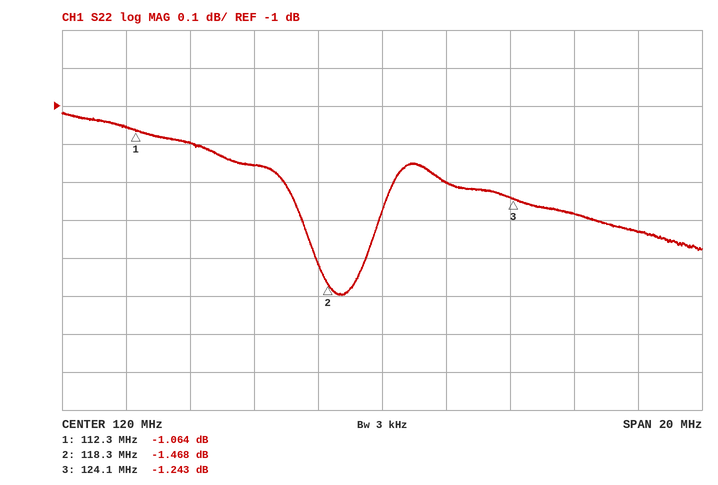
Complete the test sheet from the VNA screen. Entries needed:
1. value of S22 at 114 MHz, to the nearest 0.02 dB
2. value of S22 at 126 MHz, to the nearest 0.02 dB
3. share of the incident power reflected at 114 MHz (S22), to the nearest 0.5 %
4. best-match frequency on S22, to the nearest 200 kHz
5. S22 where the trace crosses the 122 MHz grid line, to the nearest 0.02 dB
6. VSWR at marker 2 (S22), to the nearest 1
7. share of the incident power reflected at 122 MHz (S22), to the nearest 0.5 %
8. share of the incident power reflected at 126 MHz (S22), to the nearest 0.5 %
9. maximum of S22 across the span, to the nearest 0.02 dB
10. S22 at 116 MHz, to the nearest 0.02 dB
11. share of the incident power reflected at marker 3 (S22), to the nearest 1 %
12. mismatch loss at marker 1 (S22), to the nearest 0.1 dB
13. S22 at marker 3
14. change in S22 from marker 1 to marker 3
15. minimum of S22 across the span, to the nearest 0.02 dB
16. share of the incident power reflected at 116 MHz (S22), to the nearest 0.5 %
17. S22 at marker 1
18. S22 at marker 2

-1.10 dB
-1.28 dB
77.5 %
118.8 MHz
-1.20 dB
12
76.0 %
74.5 %
-1.02 dB
-1.16 dB
75 %
6.6 dB
-1.243 dB
-0.179 dB
-1.50 dB
76.5 %
-1.064 dB
-1.468 dB
